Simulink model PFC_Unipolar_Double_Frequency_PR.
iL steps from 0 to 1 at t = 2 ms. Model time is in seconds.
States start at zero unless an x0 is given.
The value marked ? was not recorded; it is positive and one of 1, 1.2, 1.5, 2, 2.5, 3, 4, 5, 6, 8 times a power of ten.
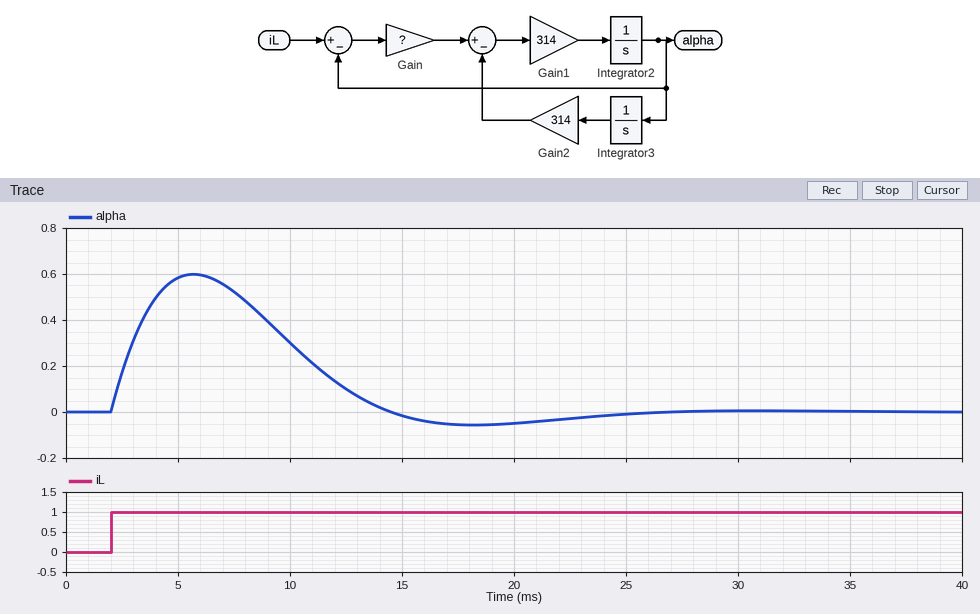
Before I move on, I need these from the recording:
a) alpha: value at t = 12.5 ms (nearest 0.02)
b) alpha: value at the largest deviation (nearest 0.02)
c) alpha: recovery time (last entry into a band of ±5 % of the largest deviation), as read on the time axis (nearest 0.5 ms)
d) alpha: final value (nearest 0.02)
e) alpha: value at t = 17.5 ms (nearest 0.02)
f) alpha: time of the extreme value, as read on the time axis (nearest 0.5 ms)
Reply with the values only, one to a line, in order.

0.10
0.60
22.5 ms
0.00
-0.06
5.5 ms
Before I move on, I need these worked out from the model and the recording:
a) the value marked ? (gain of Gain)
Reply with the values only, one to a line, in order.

1.2
